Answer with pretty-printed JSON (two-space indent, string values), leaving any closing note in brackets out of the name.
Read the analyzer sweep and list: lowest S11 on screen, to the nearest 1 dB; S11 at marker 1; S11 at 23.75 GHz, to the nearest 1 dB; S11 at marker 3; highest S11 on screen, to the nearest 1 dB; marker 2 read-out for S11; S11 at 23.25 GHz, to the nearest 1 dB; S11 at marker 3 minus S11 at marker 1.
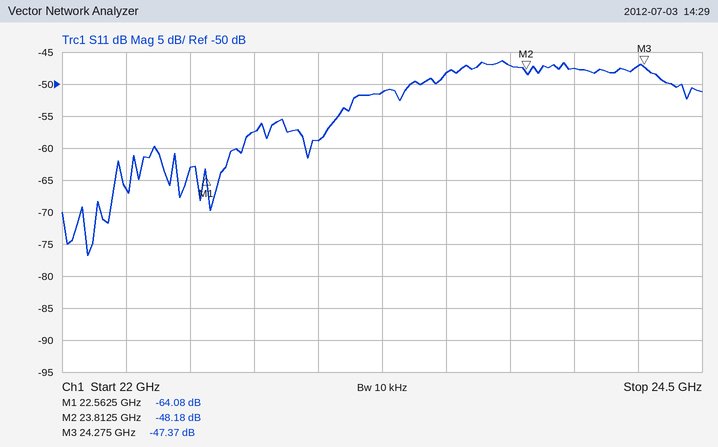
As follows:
{
  "lowest S11 on screen, to the nearest 1 dB": "-77 dB",
  "S11 at marker 1": "-64.08 dB",
  "S11 at 23.75 GHz, to the nearest 1 dB": "-47 dB",
  "S11 at marker 3": "-47.37 dB",
  "highest S11 on screen, to the nearest 1 dB": "-46 dB",
  "marker 2 read-out for S11": "-48.18 dB",
  "S11 at 23.25 GHz, to the nearest 1 dB": "-51 dB",
  "S11 at marker 3 minus S11 at marker 1": "16.71 dB"
}
